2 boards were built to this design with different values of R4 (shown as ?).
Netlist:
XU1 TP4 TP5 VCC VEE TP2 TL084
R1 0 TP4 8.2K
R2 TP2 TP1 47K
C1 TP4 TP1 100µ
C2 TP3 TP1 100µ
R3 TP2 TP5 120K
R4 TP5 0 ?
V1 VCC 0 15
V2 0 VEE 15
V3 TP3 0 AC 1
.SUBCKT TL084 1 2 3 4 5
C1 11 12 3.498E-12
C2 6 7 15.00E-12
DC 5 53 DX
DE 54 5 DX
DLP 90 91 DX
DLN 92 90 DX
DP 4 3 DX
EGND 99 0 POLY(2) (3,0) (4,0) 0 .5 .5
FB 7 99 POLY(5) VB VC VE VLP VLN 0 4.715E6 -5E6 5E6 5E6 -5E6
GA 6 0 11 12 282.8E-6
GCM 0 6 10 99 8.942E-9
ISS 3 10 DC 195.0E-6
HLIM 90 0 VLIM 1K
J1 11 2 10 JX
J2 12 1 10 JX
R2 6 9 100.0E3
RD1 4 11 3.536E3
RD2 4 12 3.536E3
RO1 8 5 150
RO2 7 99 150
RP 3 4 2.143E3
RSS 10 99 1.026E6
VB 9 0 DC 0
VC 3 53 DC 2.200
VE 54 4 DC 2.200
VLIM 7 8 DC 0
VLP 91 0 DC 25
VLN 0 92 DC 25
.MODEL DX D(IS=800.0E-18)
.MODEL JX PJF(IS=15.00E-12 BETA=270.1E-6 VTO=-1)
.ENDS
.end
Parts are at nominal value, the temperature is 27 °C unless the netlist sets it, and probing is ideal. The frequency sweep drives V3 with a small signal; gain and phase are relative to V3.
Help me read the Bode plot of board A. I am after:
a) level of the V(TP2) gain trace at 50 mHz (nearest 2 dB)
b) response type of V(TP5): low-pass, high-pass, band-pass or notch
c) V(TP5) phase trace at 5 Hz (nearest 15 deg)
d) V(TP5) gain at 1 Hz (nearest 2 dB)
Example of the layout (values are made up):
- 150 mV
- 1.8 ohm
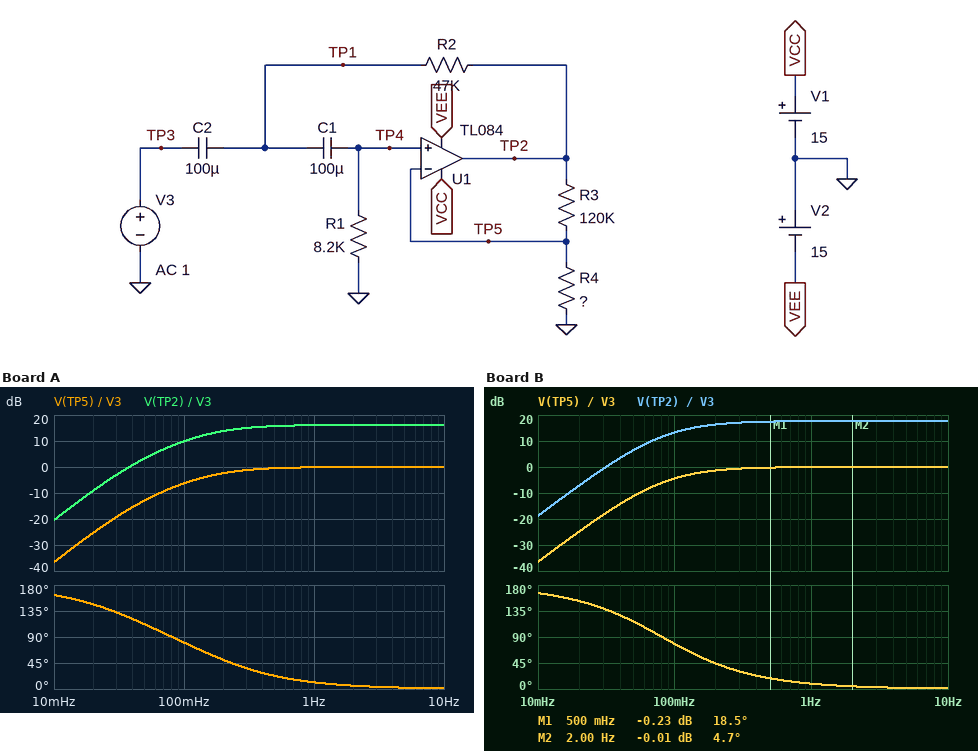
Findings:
- 4 dB
- high-pass
- 0 deg
- 0 dB
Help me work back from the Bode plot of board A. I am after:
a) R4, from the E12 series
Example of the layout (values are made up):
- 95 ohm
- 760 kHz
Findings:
- 22 kΩ
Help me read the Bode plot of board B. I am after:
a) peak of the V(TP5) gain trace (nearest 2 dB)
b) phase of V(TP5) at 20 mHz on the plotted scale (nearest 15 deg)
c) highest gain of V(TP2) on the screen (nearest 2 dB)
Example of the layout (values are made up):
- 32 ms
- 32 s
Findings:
- 0 dB
- 150 deg
- 18 dB
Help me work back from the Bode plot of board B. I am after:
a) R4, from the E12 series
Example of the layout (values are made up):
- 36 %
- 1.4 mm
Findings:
- 18 kΩ
